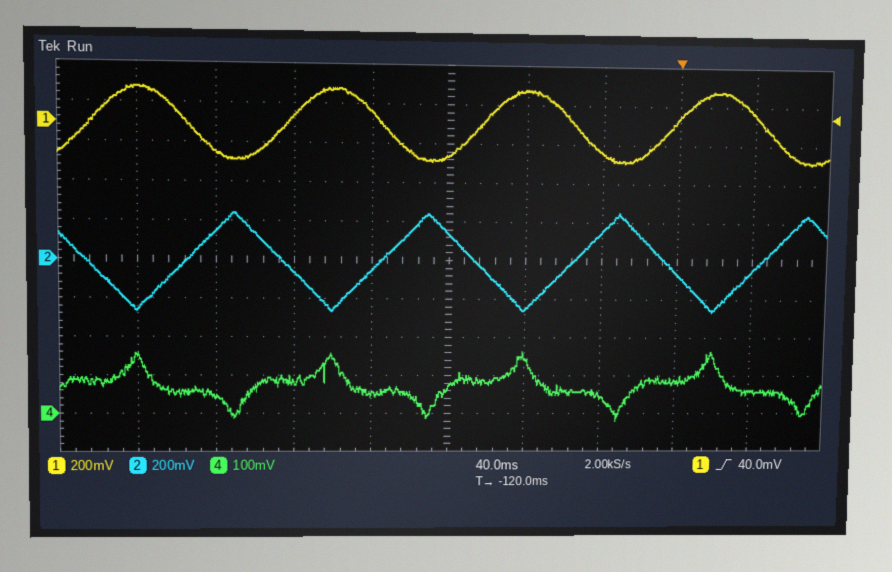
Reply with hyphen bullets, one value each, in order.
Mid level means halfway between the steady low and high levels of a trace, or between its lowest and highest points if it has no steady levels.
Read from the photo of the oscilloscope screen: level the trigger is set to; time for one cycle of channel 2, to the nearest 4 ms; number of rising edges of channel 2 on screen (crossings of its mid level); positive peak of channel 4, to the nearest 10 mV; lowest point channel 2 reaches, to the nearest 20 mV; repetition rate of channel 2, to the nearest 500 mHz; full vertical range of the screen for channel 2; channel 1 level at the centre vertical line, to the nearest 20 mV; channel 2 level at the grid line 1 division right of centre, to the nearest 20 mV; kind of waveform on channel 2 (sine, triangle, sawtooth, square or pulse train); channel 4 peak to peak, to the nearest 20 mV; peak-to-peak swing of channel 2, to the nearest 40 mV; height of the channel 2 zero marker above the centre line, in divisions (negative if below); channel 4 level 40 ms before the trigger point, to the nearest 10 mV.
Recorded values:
- 40.0 mV
- 100 ms
- 4
- 160 mV
- -260 mV
- 10.0 Hz
- 2 V
- -160 mV
- -240 mV
- triangle
- 180 mV
- 520 mV
- 0.0 div
- 50 mV
